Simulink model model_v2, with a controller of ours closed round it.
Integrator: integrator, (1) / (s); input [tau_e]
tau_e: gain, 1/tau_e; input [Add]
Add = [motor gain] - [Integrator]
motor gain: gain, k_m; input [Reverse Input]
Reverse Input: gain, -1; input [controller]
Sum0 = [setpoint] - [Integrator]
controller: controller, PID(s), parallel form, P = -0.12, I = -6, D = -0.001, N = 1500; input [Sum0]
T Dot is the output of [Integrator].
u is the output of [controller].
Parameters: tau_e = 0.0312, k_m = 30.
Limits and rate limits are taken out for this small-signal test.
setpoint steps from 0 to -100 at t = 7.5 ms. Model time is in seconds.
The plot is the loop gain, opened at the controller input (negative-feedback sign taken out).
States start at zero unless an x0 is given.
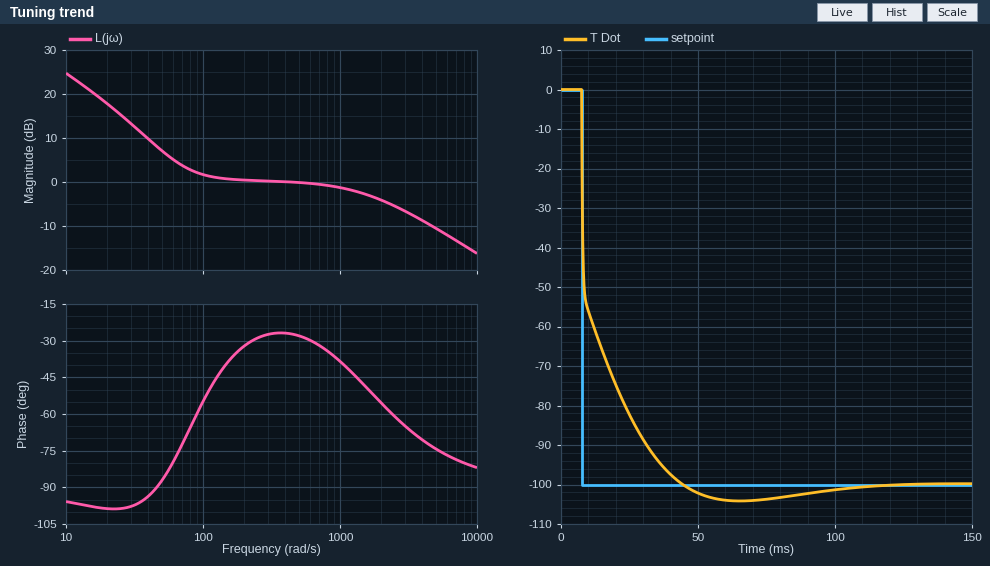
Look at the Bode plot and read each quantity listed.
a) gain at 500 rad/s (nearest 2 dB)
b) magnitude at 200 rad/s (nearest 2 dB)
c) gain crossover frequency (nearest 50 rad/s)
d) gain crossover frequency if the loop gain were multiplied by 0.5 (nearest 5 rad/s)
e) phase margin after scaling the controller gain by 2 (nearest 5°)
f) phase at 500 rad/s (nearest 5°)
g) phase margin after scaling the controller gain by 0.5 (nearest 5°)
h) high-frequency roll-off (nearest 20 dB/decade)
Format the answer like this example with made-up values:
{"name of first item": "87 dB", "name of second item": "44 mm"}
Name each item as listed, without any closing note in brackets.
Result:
{"gain at 500 rad/s": "0 dB", "magnitude at 200 rad/s": "0 dB", "gain crossover frequency": "450 rad/s", "gain crossover frequency if the loop gain were multiplied by 0.5": "55 rad/s", "phase margin after scaling the controller gain by 2": "115°", "phase at 500 rad/s": "-30°", "phase margin after scaling the controller gain by 0.5": "95°", "high-frequency roll-off": "-20 dB/decade"}
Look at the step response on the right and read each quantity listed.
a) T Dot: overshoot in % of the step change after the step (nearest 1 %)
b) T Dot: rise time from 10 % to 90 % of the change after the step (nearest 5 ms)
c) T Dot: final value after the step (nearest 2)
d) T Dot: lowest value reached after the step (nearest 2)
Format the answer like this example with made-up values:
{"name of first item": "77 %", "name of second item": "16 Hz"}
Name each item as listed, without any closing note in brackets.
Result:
{"T Dot: overshoot in % of the step change after the step": "4 %", "T Dot: rise time from 10 % to 90 % of the change after the step": "25 ms", "T Dot: final value after the step": "-100", "T Dot: lowest value reached after the step": "-104"}
